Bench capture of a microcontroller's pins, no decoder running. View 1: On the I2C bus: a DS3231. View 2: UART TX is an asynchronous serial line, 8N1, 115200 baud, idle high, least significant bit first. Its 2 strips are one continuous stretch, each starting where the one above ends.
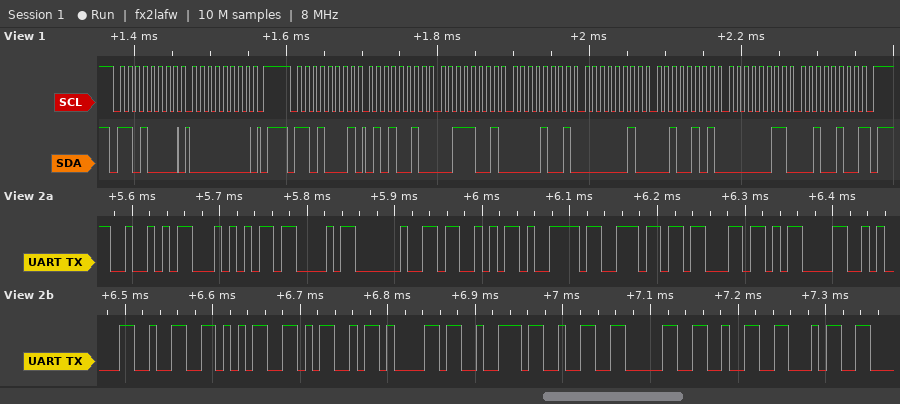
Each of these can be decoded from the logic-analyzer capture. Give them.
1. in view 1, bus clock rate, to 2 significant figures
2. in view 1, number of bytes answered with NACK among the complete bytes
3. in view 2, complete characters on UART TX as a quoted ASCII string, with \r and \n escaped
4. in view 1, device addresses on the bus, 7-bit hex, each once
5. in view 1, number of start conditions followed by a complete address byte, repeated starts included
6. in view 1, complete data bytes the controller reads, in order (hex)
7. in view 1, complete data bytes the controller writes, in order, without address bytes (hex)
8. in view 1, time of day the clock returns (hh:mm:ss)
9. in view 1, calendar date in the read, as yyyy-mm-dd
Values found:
100 kHz
1
"RTC Sync\r\n25Mar2024"
0x68
2
52 39 09 02 25 03 24
00
09:39:52
2024-03-25
